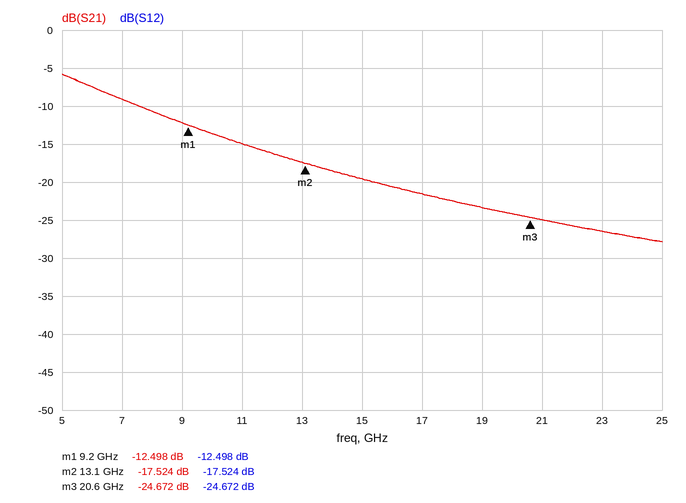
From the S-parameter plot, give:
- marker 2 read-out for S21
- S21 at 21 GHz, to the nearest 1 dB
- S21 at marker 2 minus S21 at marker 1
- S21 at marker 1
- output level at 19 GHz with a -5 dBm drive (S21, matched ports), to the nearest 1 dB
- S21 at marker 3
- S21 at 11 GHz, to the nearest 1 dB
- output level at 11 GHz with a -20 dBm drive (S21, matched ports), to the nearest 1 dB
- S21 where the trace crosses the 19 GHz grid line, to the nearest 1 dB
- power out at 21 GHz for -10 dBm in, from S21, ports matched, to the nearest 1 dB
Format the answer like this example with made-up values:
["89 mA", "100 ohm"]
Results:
["-17.524 dB", "-25 dB", "-5.026 dB", "-12.498 dB", "-28 dBm", "-24.672 dB", "-15 dB", "-35 dBm", "-23 dB", "-35 dBm"]
